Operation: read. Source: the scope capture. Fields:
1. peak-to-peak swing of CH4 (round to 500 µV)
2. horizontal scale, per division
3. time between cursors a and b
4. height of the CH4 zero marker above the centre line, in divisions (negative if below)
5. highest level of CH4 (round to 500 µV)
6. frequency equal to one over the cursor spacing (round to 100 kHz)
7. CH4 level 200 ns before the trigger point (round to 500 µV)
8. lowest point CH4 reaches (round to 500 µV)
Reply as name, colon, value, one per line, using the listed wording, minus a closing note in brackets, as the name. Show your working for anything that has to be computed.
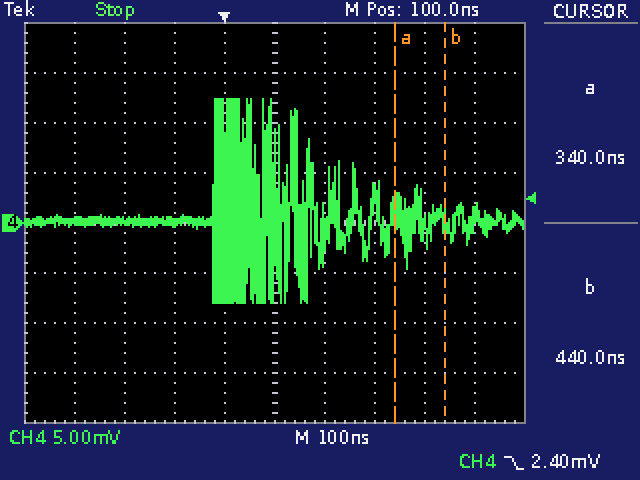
peak-to-peak swing of CH4: 12.5 mV − (-8.0 mV) = 20.5 mV
horizontal scale, per division: 100 ns
time between cursors a and b: 440 ns − (340 ns) = 100 ns
height of the CH4 zero marker above the centre line, in divisions: 0.0 div
highest level of CH4: 12.5 mV
frequency equal to one over the cursor spacing: 1 / 100 ns ≈ 10.0 MHz
CH4 level 200 ns before the trigger point: 0.0 mV
lowest point CH4 reaches: -8.0 mV
